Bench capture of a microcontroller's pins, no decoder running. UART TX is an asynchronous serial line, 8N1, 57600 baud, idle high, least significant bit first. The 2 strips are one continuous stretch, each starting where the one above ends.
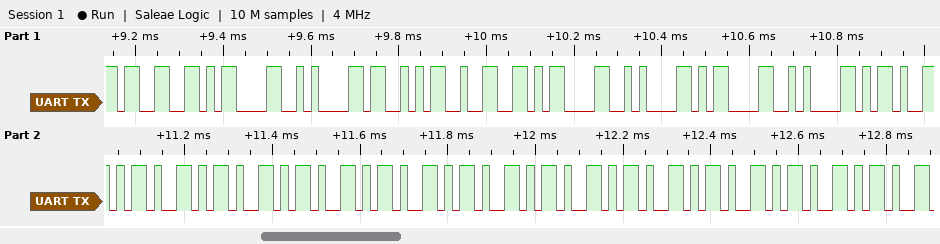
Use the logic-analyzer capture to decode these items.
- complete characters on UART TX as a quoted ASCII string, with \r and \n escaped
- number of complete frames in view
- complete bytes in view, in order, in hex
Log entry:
"3\r\nS2\r\n\r\n-----------"
20
33 0D 0A 53 32 0D 0A 0D 0A 2D 2D 2D 2D 2D 2D 2D 2D 2D 2D 2D
